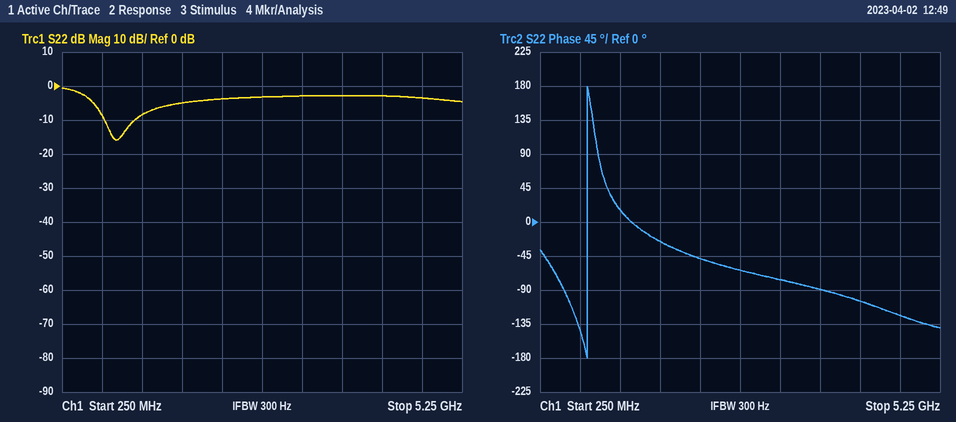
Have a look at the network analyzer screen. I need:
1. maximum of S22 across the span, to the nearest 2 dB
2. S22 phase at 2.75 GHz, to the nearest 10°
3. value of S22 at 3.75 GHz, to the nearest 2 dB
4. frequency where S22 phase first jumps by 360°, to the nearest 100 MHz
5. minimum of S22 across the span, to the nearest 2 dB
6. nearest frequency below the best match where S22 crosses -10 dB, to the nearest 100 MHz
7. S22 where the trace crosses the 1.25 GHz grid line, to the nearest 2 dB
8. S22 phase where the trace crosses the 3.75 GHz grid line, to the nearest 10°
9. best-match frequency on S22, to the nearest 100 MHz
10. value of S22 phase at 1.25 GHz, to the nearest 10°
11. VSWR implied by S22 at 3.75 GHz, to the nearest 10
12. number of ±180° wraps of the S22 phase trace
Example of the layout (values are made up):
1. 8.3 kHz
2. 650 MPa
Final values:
1. 0 dB
2. -60°
3. -2 dB
4. 800 MHz
5. -16 dB
6. 800 MHz
7. -8 dB
8. -90°
9. 900 MHz
10. 20°
11. 10
12. 1
